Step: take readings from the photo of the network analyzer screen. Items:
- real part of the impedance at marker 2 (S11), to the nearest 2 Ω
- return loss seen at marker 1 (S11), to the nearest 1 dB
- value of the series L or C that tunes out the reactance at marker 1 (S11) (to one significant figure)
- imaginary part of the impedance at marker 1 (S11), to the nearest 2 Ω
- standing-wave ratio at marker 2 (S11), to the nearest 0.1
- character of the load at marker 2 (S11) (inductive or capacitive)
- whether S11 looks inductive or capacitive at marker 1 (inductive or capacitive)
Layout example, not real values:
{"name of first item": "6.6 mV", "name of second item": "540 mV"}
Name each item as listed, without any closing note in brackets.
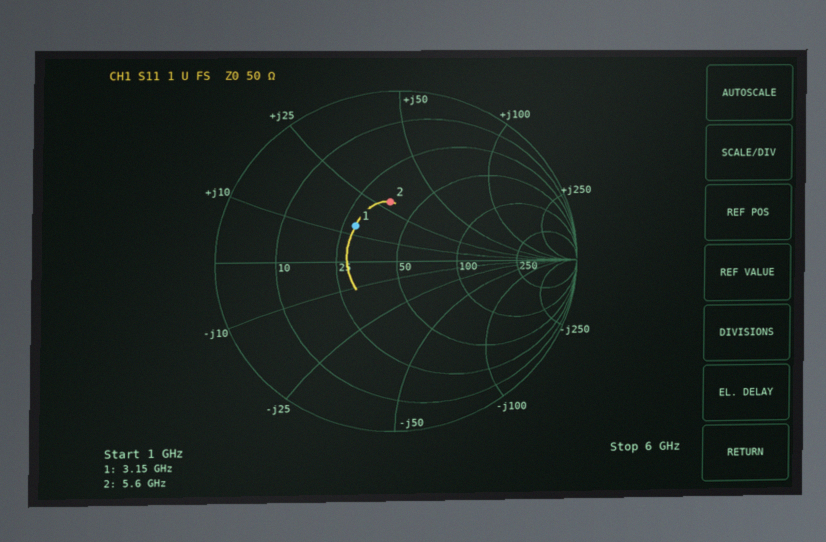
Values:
{"real part of the impedance at marker 2 (S11), to the nearest 2 Ω": "36 Ω", "return loss seen at marker 1 (S11), to the nearest 1 dB": "10 dB", "value of the series L or C that tunes out the reactance at marker 1 (S11)": "4 pF", "imaginary part of the impedance at marker 1 (S11), to the nearest 2 Ω": "+14 Ω", "standing-wave ratio at marker 2 (S11), to the nearest 0.1": "2.1", "character of the load at marker 2 (S11)": "inductive", "whether S11 looks inductive or capacitive at marker 1": "inductive"}
